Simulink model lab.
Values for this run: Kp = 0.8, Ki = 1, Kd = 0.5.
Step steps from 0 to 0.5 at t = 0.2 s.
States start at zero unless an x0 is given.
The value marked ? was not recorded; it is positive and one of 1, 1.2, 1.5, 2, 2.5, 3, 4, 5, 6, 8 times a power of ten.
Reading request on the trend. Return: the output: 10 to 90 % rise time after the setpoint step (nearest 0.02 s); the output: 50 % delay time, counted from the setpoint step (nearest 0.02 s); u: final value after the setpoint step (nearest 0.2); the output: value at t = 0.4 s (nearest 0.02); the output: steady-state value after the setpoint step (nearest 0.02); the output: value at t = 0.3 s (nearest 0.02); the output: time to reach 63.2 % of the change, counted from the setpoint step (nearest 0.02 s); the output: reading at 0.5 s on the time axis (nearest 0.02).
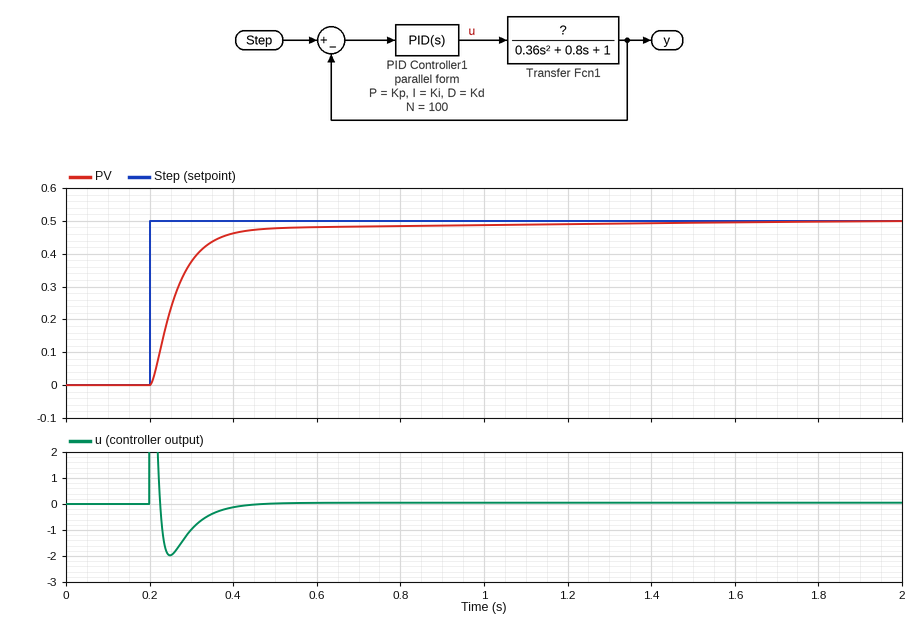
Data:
0.16 s
0.06 s
0.0
0.46
0.50
0.38
0.08 s
0.48
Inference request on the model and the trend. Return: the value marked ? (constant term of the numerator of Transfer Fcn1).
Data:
10
